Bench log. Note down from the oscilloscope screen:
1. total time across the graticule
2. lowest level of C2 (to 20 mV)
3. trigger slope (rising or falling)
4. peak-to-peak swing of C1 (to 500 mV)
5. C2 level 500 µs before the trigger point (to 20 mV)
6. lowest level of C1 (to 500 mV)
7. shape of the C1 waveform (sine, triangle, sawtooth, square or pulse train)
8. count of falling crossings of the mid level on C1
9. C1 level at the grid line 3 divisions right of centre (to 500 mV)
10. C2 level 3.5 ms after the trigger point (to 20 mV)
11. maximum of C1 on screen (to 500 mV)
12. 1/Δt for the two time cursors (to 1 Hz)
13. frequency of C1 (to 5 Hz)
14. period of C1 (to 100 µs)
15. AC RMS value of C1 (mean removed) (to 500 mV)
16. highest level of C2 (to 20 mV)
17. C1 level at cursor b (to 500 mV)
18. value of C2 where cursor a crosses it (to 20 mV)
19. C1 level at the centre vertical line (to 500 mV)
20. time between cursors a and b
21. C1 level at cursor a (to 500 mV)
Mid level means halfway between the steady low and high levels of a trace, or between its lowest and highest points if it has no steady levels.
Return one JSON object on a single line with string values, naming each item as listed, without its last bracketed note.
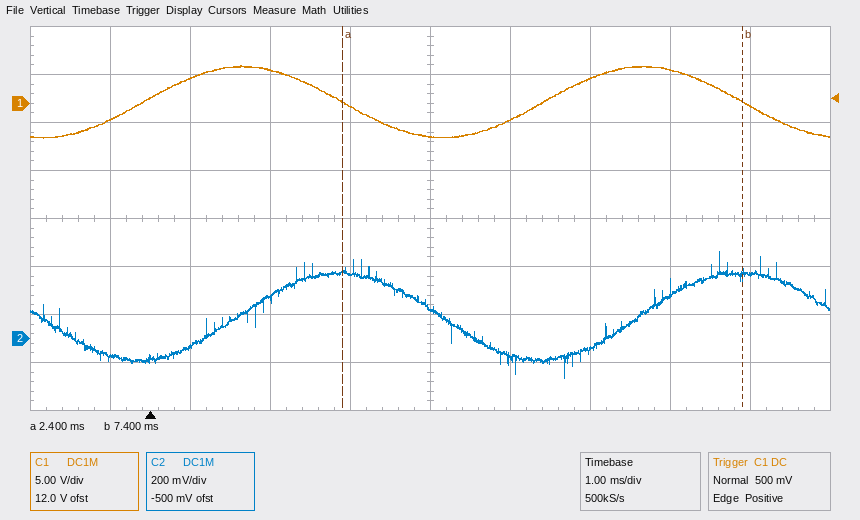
{"total time across the graticule": "10 ms", "lowest level of C2": "-160 mV", "trigger slope": "rising", "peak-to-peak swing of C1": "7.5 V", "C2 level 500 µs before the trigger point": "-80 mV", "lowest level of C1": "-3.5 V", "shape of the C1 waveform": "sine", "count of falling crossings of the mid level on C1": "2", "C1 level at the grid line 3 divisions right of centre": "3.5 V", "C2 level 3.5 ms after the trigger point": "120 mV", "maximum of C1 on screen": "4.0 V", "1/Δt for the two time cursors": "200 Hz", "frequency of C1": "200 Hz", "period of C1": "5.0 ms", "AC RMS value of C1 (mean removed)": "2.5 V", "highest level of C2": "360 mV", "C1 level at cursor b": "0.0 V", "value of C2 where cursor a crosses it": "280 mV", "C1 level at the centre vertical line": "-3.5 V", "time between cursors a and b": "5.0 ms", "C1 level at cursor a": "0.0 V"}
